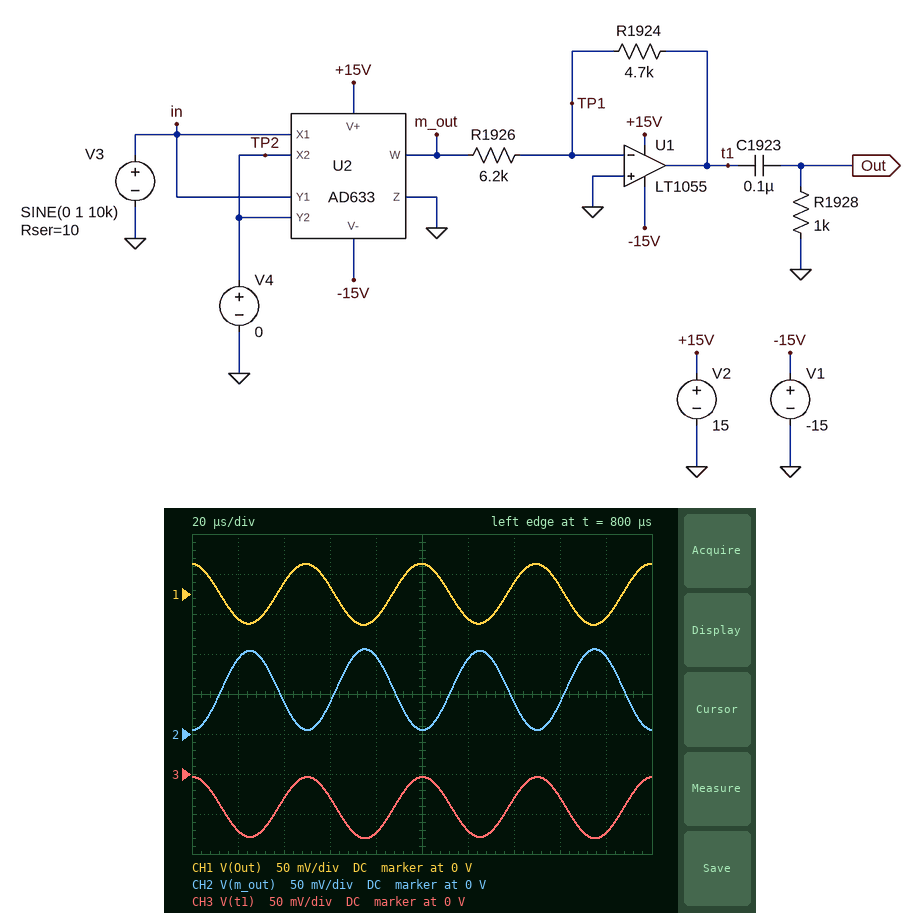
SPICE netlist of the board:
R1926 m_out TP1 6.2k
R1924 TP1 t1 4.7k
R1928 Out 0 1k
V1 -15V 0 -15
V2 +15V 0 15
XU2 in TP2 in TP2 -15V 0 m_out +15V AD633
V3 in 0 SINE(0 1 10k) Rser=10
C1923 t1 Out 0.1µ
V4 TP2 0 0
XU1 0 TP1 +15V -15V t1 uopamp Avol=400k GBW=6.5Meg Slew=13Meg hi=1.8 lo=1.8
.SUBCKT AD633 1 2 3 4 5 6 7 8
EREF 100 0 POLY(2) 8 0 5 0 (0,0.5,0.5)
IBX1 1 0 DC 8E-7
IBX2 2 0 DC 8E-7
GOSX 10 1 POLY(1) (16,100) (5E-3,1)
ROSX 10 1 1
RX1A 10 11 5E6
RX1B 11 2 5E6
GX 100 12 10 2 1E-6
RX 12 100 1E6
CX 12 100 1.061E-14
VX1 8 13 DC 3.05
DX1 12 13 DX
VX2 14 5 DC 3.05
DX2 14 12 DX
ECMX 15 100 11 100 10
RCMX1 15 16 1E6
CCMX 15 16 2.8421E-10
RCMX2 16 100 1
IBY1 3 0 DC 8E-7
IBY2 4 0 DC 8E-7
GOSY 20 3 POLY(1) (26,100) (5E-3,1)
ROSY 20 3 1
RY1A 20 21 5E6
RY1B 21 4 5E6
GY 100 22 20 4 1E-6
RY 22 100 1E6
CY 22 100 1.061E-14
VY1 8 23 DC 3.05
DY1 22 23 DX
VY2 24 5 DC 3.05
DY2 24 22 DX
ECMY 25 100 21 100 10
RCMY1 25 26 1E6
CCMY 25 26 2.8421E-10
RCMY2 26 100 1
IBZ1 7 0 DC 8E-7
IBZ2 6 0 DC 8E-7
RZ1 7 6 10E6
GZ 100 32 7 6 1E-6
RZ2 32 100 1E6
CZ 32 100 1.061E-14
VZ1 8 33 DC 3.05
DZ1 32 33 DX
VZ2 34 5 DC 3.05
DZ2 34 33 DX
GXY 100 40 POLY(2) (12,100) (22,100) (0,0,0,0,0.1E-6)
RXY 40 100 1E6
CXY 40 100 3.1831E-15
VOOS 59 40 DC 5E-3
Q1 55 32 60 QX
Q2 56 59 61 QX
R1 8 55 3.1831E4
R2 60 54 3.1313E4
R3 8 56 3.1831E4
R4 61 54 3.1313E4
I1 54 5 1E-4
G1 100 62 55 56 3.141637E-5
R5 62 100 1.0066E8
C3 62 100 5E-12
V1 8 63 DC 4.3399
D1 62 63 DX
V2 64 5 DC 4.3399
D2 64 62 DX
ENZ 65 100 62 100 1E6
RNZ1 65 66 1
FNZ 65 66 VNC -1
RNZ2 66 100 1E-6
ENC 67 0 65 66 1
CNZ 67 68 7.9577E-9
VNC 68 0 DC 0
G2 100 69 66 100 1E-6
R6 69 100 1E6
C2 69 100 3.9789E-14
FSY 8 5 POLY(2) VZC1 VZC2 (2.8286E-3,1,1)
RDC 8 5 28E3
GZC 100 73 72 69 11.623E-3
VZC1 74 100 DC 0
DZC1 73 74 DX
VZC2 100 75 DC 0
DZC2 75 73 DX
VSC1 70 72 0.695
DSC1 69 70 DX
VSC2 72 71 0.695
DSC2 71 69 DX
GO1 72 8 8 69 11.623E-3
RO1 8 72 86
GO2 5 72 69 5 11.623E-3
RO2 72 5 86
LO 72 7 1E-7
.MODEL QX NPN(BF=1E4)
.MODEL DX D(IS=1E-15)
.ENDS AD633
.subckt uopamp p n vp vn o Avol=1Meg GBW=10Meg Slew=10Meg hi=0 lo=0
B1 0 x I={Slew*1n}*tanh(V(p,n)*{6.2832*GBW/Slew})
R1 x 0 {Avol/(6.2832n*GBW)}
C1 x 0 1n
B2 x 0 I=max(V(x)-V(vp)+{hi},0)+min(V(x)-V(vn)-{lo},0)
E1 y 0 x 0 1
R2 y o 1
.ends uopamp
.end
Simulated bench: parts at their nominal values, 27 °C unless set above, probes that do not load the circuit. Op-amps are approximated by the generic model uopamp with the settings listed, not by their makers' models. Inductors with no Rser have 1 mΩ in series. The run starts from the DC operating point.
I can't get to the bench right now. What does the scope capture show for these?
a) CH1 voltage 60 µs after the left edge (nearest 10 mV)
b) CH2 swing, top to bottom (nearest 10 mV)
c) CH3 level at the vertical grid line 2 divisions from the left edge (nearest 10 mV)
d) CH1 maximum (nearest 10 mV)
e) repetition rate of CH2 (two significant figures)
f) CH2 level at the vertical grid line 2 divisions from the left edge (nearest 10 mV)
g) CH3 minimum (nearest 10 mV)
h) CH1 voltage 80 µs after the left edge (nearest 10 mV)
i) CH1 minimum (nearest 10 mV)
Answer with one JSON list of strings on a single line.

["10 mV", "100 mV", "-30 mV", "40 mV", "20 kHz", "40 mV", "-80 mV", "-30 mV", "-40 mV"]
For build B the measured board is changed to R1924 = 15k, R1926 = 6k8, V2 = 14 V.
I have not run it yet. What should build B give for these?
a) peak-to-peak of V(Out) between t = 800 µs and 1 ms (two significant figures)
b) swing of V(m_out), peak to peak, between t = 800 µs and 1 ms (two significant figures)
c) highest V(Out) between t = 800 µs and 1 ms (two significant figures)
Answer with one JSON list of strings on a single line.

["220 mV", "100 mV", "110 mV"]
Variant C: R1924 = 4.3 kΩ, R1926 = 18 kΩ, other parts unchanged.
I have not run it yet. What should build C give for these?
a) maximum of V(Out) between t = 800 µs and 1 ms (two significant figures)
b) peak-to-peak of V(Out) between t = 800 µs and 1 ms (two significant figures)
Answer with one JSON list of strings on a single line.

["12 mV", "24 mV"]
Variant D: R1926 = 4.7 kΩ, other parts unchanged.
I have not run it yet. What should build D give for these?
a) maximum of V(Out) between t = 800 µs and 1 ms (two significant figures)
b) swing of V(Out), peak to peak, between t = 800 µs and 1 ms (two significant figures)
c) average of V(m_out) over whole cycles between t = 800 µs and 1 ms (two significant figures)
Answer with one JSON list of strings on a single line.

["50 mV", "100 mV", "55 mV"]
